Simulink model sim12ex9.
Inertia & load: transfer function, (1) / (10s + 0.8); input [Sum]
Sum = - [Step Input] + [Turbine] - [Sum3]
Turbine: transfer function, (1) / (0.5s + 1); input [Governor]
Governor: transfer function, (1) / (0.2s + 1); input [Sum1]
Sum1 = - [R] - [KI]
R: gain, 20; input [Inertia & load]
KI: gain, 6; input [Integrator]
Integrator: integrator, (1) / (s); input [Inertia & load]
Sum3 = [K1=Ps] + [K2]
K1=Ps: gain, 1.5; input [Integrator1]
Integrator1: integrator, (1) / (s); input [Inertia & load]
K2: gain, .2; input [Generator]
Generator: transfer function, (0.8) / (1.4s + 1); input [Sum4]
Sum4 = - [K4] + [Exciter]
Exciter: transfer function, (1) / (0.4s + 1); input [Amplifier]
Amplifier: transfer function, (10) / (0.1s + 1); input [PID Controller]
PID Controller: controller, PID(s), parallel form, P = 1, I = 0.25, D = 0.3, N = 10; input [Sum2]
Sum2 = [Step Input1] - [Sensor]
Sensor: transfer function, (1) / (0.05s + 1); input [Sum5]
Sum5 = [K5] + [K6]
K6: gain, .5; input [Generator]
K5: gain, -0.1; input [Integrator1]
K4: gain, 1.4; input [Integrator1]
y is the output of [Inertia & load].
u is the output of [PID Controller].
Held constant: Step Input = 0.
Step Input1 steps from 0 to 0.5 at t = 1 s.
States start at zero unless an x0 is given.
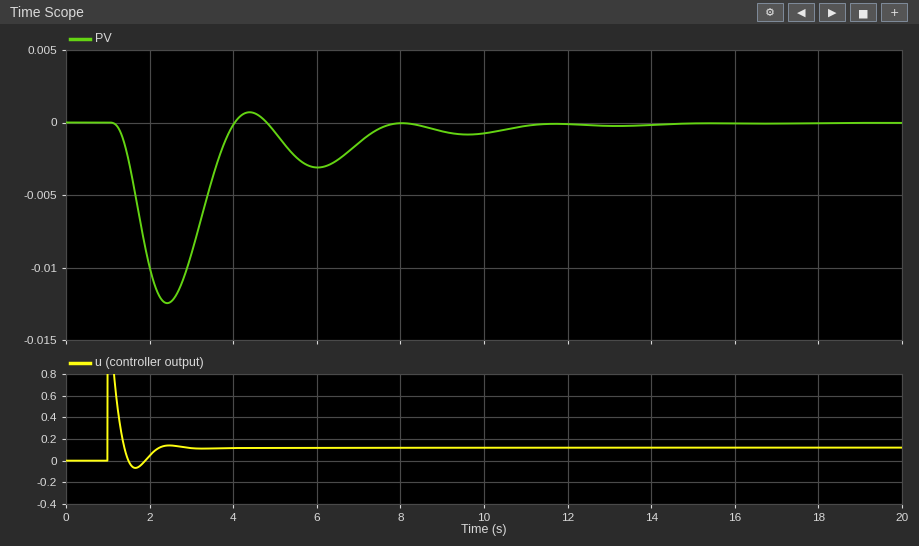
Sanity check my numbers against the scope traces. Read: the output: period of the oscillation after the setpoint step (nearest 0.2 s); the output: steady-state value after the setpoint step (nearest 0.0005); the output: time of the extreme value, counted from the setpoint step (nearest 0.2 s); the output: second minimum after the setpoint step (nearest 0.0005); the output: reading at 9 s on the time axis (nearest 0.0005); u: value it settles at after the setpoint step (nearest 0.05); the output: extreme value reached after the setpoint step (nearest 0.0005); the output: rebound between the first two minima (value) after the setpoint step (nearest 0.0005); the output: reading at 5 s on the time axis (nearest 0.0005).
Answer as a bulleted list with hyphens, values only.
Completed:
- 3.6 s
- 0.0000
- 1.4 s
- -0.0030
- -0.0005
- 0.10
- -0.0125
- 0.0005
- -0.0005
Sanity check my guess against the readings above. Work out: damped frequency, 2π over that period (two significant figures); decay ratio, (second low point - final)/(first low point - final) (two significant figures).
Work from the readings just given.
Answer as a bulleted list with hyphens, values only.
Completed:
- 1.7 rad/s
- 0.24
